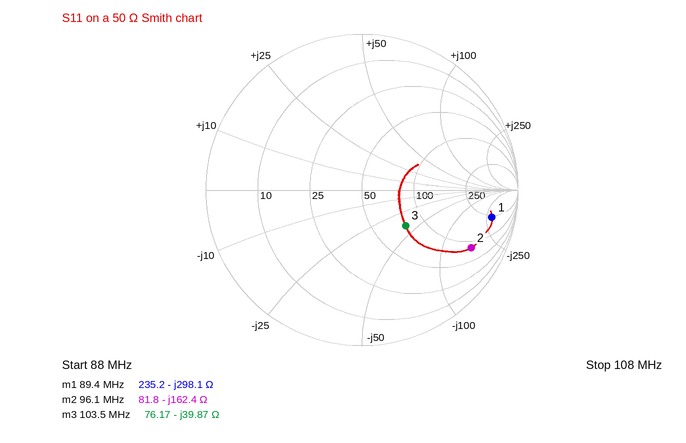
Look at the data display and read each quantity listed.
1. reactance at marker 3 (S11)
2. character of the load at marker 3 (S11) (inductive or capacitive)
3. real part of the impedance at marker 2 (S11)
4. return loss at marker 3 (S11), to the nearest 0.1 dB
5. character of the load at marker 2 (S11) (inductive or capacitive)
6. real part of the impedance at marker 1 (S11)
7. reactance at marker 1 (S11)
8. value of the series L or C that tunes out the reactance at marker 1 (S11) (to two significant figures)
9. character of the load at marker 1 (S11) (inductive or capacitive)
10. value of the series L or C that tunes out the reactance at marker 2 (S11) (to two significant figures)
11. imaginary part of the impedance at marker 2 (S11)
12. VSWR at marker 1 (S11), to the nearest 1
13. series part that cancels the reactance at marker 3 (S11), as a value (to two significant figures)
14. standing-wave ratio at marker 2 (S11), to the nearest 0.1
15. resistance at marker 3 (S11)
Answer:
-39.87 Ω
capacitive
81.8 Ω
8.9 dB
capacitive
235.2 Ω
-298.1 Ω
530 nH
capacitive
270 nH
-162.4 Ω
12
61 nH
8.6
76.17 Ω
